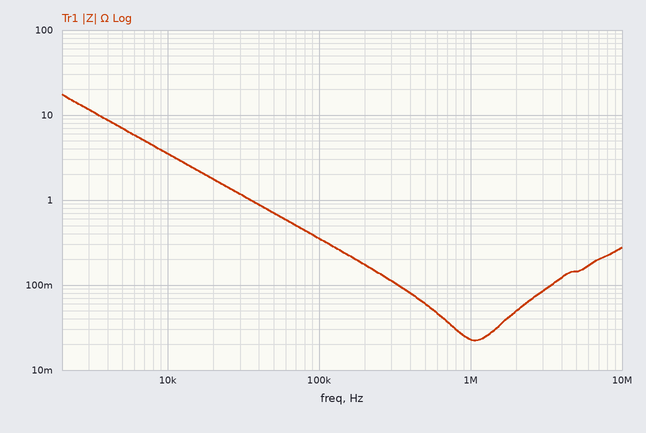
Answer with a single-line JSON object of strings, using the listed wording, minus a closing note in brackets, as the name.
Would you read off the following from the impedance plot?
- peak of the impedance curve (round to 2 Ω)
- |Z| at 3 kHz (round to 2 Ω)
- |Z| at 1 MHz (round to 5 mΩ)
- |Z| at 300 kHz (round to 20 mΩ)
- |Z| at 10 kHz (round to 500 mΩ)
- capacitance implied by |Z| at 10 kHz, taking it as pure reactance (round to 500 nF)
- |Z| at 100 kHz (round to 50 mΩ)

{"peak of the impedance curve": "18 Ω", "|Z| at 3 kHz": "12 Ω", "|Z| at 1 MHz": "25 mΩ", "|Z| at 300 kHz": "120 mΩ", "|Z| at 10 kHz": "3.5 Ω", "capacitance implied by |Z| at 10 kHz, taking it as pure reactance": "4.5 µF", "|Z| at 100 kHz": "350 mΩ"}
